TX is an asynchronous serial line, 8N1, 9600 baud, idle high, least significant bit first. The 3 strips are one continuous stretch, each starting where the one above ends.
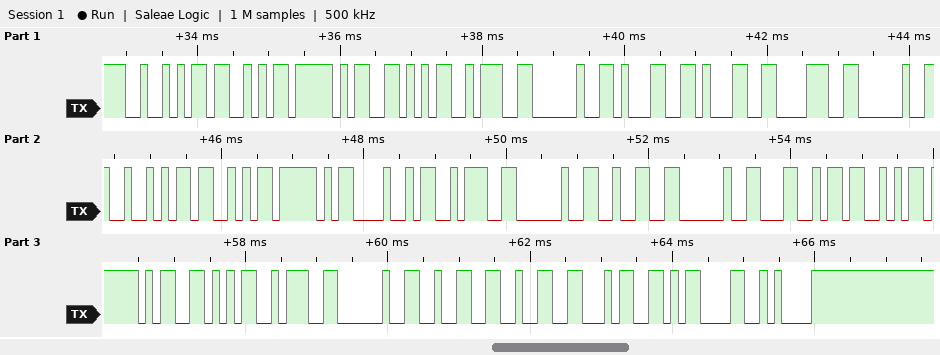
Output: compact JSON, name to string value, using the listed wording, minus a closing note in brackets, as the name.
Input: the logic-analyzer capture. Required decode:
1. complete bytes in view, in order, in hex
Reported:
{"complete bytes in view, in order, in hex": "52 53 5F 56 3A 20 31 31 38 20 52 53 5F 48 3A 20 32 20 4C 53 5F 56 3A 20 32 32 34 0D 0A"}
